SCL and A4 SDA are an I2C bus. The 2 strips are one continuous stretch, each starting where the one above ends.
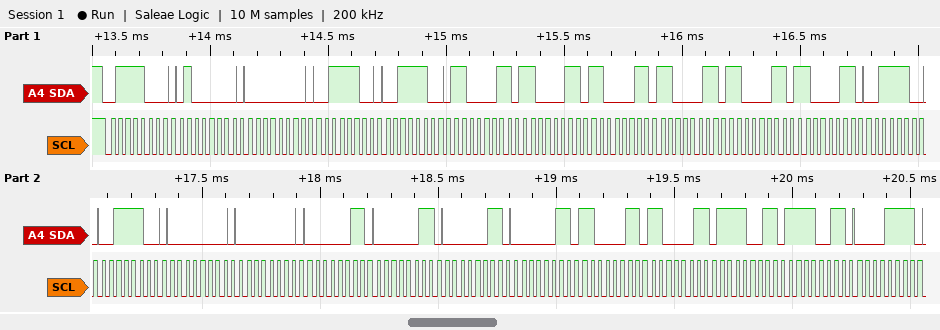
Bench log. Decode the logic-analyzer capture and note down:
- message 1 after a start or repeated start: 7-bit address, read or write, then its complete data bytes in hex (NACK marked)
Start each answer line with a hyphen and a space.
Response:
- 0x3C write: 40 00 3C 3C C3 C3 C3 C3 C3 C3 3C 3C 00 00 03 03 03 03 C3 C3 F3 F3 0F
